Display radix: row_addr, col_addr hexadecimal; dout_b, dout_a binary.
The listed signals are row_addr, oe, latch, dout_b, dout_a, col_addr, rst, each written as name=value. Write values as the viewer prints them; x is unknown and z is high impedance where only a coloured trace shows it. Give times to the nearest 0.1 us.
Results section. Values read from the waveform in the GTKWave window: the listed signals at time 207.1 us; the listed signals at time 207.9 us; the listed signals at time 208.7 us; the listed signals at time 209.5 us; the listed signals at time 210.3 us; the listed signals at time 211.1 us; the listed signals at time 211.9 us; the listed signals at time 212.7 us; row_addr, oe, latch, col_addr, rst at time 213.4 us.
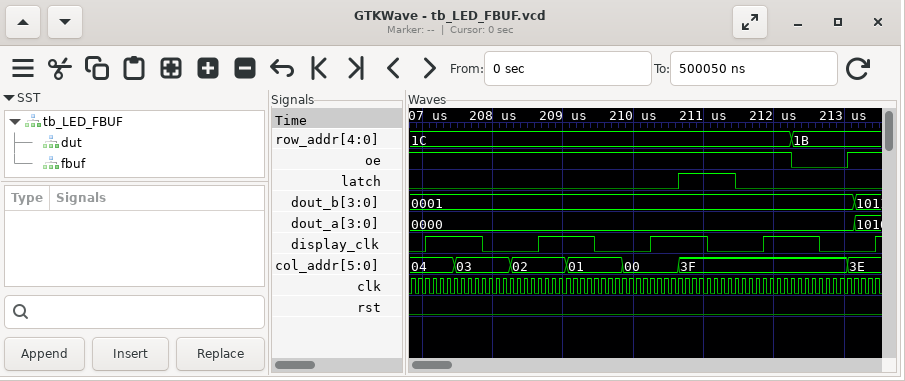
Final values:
row_addr=1C, oe=1, latch=0, dout_b=0001, dout_a=0000, col_addr=04, rst=0
row_addr=1C, oe=1, latch=0, dout_b=0001, dout_a=0000, col_addr=03, rst=0
row_addr=1C, oe=1, latch=0, dout_b=0001, dout_a=0000, col_addr=02, rst=0
row_addr=1C, oe=1, latch=0, dout_b=0001, dout_a=0000, col_addr=01, rst=0
row_addr=1C, oe=1, latch=0, dout_b=0001, dout_a=0000, col_addr=00, rst=0
row_addr=1C, oe=1, latch=1, dout_b=0001, dout_a=0000, col_addr=3F, rst=0
row_addr=1C, oe=1, latch=0, dout_b=0001, dout_a=0000, col_addr=3F, rst=0
row_addr=1B, oe=0, latch=0, dout_b=0001, dout_a=0000, col_addr=3F, rst=0
row_addr=1B, oe=1, latch=0, col_addr=3E, rst=0
